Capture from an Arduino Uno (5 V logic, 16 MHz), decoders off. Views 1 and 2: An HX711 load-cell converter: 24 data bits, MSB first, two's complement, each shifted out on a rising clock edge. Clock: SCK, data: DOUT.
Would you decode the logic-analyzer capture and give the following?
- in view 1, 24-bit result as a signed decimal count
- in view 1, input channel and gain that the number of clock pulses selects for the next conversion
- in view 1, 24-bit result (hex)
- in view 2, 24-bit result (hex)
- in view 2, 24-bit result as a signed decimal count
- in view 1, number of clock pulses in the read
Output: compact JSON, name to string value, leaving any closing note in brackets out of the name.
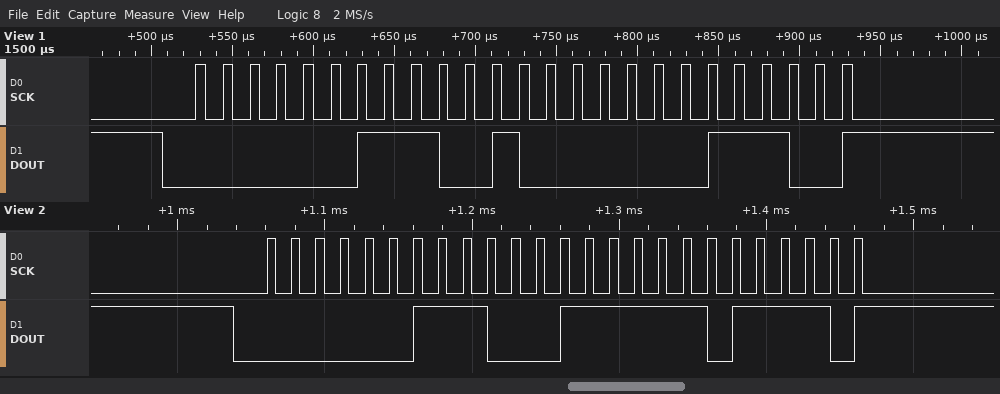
{"in view 1, 24-bit result as a signed decimal count": "233500", "in view 1, input channel and gain that the number of clock pulses selects for the next conversion": "channel A, gain 128", "in view 1, 24-bit result": "0x03901C", "in view 2, 24-bit result": "0x038FDE", "in view 2, 24-bit result as a signed decimal count": "233438", "in view 1, number of clock pulses in the read": "25"}
